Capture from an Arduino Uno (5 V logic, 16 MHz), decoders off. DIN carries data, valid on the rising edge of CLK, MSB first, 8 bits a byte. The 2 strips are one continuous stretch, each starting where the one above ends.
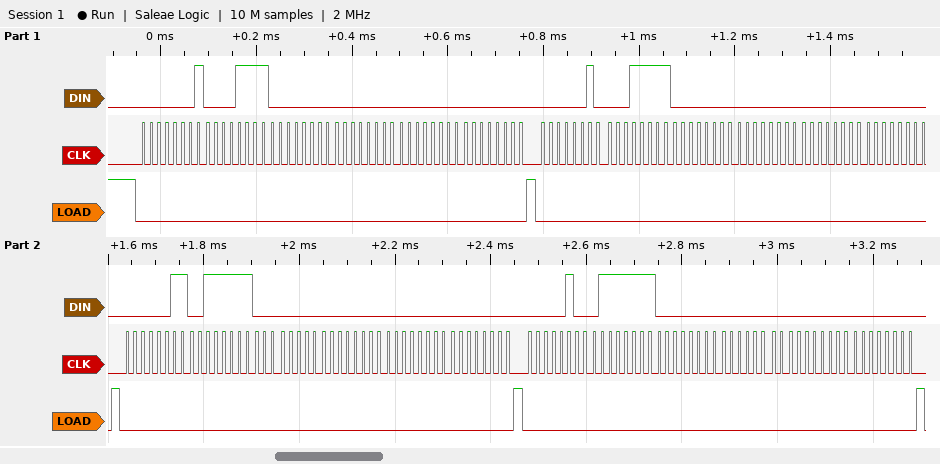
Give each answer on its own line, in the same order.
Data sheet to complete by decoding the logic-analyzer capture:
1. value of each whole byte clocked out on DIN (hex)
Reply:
01 0F 00 00 00 00 02 1F 00 00 00 00 03 3F 00 00 00 00 04 7F 00 00 00 00
